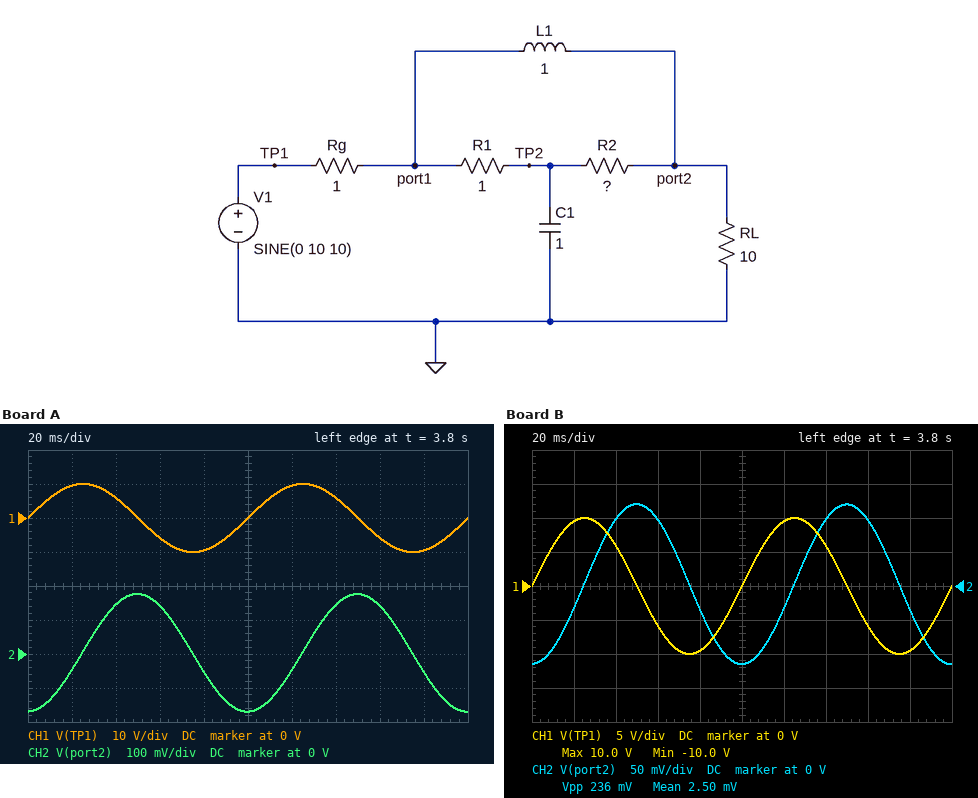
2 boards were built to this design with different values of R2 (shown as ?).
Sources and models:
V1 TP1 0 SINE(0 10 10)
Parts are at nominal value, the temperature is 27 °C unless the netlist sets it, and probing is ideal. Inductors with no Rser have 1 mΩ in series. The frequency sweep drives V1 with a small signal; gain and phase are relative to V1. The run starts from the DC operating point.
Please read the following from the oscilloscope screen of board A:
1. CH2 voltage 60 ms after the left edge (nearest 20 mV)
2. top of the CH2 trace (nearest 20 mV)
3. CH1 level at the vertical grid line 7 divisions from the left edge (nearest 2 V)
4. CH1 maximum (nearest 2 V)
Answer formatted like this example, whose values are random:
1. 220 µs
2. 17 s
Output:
1. 140 mV
2. 180 mV
3. 6 V
4. 10 V
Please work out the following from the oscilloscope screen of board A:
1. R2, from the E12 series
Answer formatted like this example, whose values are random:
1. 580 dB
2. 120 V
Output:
1. 1.5 Ω
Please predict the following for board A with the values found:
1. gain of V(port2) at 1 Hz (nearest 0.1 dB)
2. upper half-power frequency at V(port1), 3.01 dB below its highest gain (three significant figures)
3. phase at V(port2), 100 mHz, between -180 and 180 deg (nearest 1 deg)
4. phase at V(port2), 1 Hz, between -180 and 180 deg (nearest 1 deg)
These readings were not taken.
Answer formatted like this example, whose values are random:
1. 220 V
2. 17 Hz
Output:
1. -15.5 dB
2. 116 mHz
3. -30 deg
4. -78 deg
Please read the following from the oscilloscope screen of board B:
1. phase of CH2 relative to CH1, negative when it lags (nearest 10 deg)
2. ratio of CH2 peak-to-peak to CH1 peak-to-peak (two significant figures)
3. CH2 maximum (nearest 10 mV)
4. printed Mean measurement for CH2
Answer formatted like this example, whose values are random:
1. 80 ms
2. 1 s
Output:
1. -90 deg
2. 0.012
3. 120 mV
4. 2.50 mV
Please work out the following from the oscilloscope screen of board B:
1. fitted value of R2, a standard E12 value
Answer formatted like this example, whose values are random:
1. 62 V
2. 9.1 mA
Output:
1. 0.56 Ω
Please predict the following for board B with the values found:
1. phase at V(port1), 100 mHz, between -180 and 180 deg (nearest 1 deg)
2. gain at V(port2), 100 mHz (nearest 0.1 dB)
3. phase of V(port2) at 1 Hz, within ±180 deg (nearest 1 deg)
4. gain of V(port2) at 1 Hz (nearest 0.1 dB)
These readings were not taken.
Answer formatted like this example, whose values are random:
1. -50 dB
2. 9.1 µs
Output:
1. -24 deg
2. -2.0 dB
3. -84 deg
4. -18.6 dB
